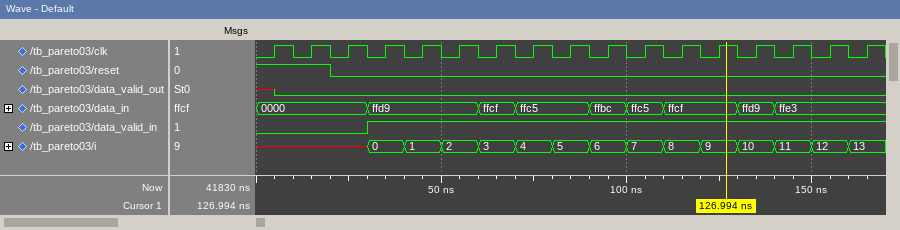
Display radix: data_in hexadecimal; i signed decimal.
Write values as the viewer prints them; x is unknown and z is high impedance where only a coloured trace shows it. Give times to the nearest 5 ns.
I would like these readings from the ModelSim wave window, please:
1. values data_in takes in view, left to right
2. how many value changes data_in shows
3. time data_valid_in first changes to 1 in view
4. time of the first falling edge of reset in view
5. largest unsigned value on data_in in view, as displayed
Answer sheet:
0000, ffd9, ffcf, ffc5, ffbc, ffc5, ffcf, ffd9, ffe3
8
30 ns
20 ns
ffe3
